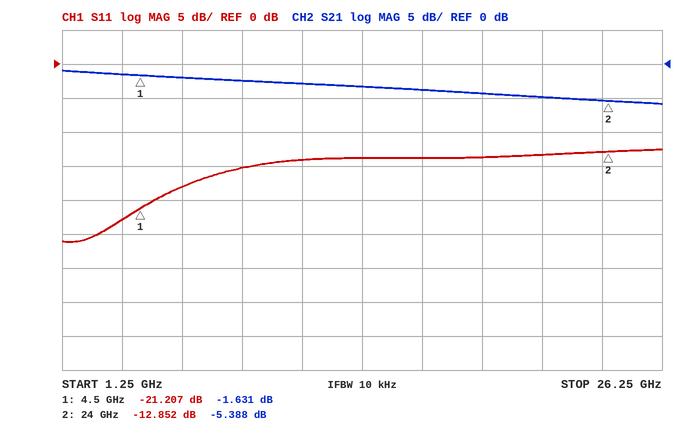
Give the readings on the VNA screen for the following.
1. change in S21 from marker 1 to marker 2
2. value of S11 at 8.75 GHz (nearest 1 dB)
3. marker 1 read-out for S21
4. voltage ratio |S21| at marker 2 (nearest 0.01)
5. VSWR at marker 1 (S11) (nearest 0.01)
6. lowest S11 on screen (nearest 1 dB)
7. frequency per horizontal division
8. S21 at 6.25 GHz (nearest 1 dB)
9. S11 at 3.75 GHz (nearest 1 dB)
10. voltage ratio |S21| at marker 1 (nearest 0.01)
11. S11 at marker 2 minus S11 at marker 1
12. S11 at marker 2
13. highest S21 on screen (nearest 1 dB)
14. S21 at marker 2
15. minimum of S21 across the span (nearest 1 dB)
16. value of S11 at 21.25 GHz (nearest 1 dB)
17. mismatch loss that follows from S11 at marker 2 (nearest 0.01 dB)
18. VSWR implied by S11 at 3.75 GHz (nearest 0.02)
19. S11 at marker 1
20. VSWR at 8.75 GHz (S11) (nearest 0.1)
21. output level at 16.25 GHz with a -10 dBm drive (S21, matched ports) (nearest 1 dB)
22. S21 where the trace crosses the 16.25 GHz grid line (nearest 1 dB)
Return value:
-3.757 dB
-15 dB
-1.631 dB
0.54
1.19
-26 dB
2.5 GHz
-2 dB
-23 dB
0.83
8.355 dB
-12.852 dB
-1 dB
-5.388 dB
-6 dB
-13 dB
0.23 dB
1.16
-21.207 dB
1.4
-14 dBm
-4 dB
